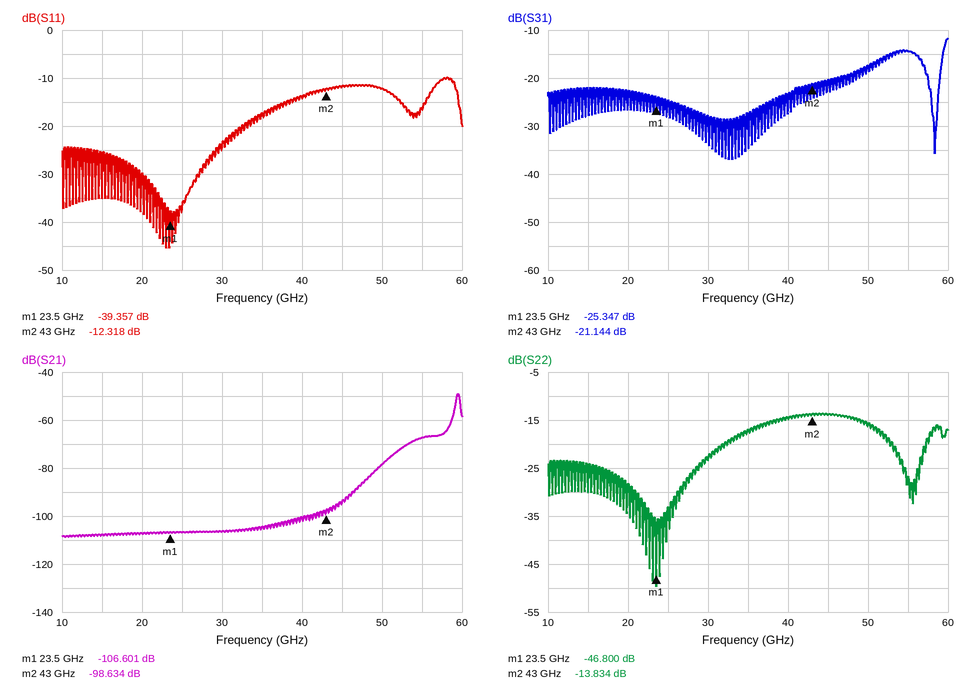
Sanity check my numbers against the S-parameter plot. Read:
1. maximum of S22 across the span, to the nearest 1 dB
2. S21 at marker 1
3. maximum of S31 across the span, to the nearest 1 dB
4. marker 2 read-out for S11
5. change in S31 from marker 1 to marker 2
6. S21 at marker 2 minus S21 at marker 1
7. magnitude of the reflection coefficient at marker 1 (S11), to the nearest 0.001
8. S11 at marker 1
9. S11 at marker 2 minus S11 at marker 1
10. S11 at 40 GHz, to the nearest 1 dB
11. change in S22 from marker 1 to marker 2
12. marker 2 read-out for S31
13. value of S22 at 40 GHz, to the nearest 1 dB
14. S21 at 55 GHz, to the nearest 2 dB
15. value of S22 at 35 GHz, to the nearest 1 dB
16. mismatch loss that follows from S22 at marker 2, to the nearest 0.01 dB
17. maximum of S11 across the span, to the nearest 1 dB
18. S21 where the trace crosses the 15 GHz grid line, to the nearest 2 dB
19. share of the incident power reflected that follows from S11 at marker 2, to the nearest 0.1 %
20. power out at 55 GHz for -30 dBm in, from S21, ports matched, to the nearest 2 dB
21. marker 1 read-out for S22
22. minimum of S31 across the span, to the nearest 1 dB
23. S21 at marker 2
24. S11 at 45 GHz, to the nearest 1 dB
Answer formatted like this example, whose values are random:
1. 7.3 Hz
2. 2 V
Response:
1. -14 dB
2. -106.601 dB
3. -12 dB
4. -12.318 dB
5. 4.203 dB
6. 7.967 dB
7. 0.011
8. -39.357 dB
9. 27.039 dB
10. -14 dB
11. 32.966 dB
12. -21.144 dB
13. -15 dB
14. -68 dB
15. -17 dB
16. 0.18 dB
17. -10 dB
18. -108 dB
19. 5.9 %
20. -98 dBm
21. -46.800 dB
22. -37 dB
23. -98.634 dB
24. -12 dB
